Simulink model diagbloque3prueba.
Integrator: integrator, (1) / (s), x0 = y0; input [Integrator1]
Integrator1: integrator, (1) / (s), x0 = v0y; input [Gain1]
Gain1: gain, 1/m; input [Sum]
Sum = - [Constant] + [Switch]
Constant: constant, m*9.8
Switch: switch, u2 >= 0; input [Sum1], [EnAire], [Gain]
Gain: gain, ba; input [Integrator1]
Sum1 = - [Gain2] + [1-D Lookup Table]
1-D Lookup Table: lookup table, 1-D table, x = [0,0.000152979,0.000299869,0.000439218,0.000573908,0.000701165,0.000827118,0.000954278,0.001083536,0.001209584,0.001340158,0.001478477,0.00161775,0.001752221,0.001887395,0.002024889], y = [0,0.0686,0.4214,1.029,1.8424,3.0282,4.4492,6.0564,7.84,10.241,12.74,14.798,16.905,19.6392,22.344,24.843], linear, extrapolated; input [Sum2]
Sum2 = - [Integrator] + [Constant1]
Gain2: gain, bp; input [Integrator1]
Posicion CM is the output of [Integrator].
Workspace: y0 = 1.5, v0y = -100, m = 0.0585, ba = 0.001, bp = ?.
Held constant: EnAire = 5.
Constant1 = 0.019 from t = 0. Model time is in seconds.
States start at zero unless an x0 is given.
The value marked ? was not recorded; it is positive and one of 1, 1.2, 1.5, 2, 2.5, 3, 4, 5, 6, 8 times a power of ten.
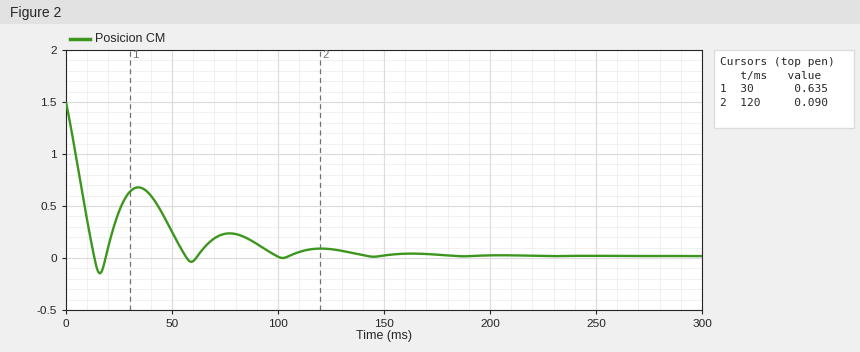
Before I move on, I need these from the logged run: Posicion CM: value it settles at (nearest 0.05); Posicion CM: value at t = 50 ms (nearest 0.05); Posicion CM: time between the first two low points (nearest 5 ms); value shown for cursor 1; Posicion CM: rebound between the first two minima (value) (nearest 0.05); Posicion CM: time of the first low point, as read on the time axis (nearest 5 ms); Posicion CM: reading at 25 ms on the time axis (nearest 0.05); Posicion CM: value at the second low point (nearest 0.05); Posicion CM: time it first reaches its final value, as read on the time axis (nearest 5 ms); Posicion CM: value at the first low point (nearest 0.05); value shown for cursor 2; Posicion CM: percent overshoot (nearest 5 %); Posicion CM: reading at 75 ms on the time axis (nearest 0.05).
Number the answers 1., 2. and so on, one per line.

1. 0.00
2. 0.25
3. 45 ms
4. 0.635
5. 0.70
6. 15 ms
7. 0.45
8. -0.05
9. 15 ms
10. -0.15
11. 0.090
12. 10 %
13. 0.25
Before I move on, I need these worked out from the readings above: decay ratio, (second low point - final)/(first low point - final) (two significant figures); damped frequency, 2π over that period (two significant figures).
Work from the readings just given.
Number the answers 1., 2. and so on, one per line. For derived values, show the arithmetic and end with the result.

1. (-0.05 - 0) / (-0.15 - 0) = 0.33
2. 2π / 45 = 0.14 rad/ms
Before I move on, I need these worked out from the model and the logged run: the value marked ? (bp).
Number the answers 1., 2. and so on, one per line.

1. 3
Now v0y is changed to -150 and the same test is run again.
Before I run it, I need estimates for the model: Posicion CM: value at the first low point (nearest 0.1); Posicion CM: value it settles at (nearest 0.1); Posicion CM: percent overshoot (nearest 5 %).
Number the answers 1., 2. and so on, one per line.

1. -0.2
2. 0.0
3. 15 %
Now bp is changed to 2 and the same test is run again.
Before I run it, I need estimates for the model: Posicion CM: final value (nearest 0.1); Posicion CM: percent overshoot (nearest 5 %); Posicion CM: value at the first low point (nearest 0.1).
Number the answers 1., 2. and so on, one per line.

1. 0.0
2. 15 %
3. -0.2
